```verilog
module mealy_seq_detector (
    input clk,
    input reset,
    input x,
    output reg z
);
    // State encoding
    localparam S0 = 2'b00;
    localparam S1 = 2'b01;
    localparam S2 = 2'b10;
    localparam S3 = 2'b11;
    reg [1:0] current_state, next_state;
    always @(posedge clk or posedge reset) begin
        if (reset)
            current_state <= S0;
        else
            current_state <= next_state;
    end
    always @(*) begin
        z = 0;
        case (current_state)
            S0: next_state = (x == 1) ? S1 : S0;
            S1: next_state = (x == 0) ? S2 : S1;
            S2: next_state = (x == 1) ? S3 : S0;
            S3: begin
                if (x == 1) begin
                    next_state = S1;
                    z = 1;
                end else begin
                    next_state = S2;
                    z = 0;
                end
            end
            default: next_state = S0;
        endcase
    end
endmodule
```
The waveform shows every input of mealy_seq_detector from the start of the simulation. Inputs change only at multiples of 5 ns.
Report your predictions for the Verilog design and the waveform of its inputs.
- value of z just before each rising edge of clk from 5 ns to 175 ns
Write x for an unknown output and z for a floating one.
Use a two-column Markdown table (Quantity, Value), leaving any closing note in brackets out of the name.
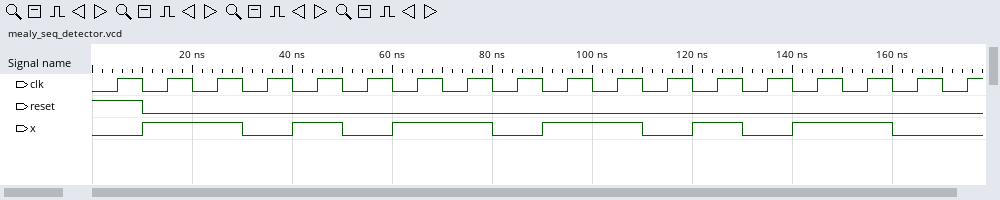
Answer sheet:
| Quantity | Value |
|---|---|
| value of z just before each rising edge of clk from 5 ns to 175 ns | 0 0 0 0 0 0 0 1 0 0 1 0 0 0 0 1 0 0 |
